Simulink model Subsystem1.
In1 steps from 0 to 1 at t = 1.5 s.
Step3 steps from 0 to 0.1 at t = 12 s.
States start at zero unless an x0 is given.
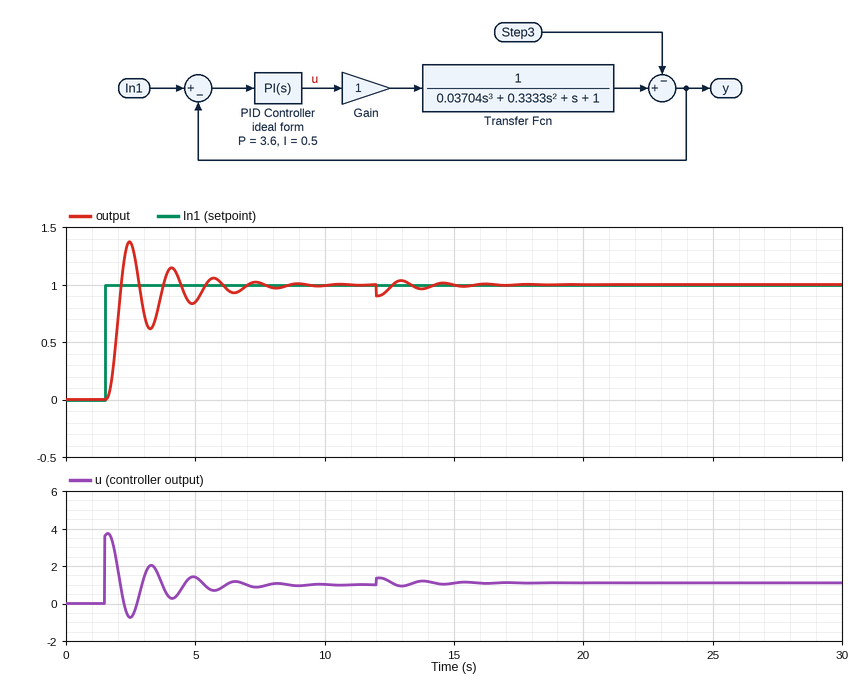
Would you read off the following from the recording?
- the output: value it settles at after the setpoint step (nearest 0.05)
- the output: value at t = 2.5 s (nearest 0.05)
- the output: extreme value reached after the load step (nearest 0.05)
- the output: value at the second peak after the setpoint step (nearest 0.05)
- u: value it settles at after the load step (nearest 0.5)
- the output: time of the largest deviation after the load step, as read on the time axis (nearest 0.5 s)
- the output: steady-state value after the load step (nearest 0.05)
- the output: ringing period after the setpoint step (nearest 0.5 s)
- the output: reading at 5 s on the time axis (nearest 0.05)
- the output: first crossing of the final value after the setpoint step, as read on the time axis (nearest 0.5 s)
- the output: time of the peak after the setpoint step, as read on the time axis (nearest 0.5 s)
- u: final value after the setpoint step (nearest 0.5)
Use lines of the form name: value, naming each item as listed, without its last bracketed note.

the output: value it settles at after the setpoint step: 1.00
the output: value at t = 2.5 s: 1.35
the output: extreme value reached after the load step: 0.90
the output: value at the second peak after the setpoint step: 1.15
u: value it settles at after the load step: 1.0
the output: time of the largest deviation after the load step, as read on the time axis: 12.0 s
the output: steady-state value after the load step: 1.00
the output: ringing period after the setpoint step: 1.5 s
the output: reading at 5 s on the time axis: 0.85
the output: first crossing of the final value after the setpoint step, as read on the time axis: 2.0 s
the output: time of the peak after the setpoint step, as read on the time axis: 2.5 s
u: final value after the setpoint step: 1.0
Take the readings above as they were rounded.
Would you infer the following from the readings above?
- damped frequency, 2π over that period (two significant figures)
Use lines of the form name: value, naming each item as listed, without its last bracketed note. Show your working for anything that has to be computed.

damped frequency, 2π over that period: 2π / 1.5 = 4.2 rad/s
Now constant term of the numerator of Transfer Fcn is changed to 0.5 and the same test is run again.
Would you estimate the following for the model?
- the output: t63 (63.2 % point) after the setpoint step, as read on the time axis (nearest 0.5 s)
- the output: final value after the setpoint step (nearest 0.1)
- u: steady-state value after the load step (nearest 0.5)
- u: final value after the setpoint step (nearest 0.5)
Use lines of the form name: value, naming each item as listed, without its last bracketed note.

the output: t63 (63.2 % point) after the setpoint step, as read on the time axis: 2.0 s
the output: final value after the setpoint step: 1.0
u: steady-state value after the load step: 2.0
u: final value after the setpoint step: 2.0
